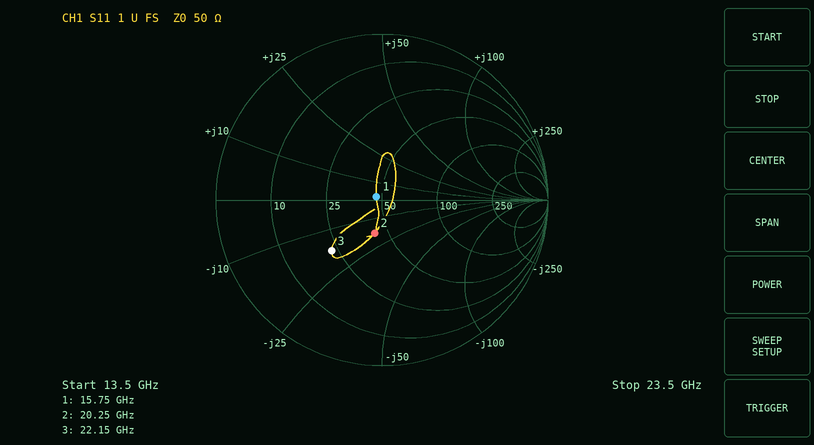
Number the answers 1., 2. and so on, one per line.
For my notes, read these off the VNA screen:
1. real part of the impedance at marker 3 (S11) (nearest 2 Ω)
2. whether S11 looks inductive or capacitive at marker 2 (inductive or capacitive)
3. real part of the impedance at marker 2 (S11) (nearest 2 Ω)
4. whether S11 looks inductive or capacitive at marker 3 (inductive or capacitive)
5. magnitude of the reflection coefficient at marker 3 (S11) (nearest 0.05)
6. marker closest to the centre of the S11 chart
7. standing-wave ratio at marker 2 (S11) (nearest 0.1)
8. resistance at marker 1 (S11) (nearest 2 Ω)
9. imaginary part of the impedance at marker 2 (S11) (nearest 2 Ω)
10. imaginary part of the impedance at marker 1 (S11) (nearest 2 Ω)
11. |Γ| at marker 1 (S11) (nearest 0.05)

1. 22 Ω
2. capacitive
3. 42 Ω
4. capacitive
5. 0.45
6. marker 1
7. 1.5
8. 46 Ω
9. -18 Ω
10. +2 Ω
11. 0.05
